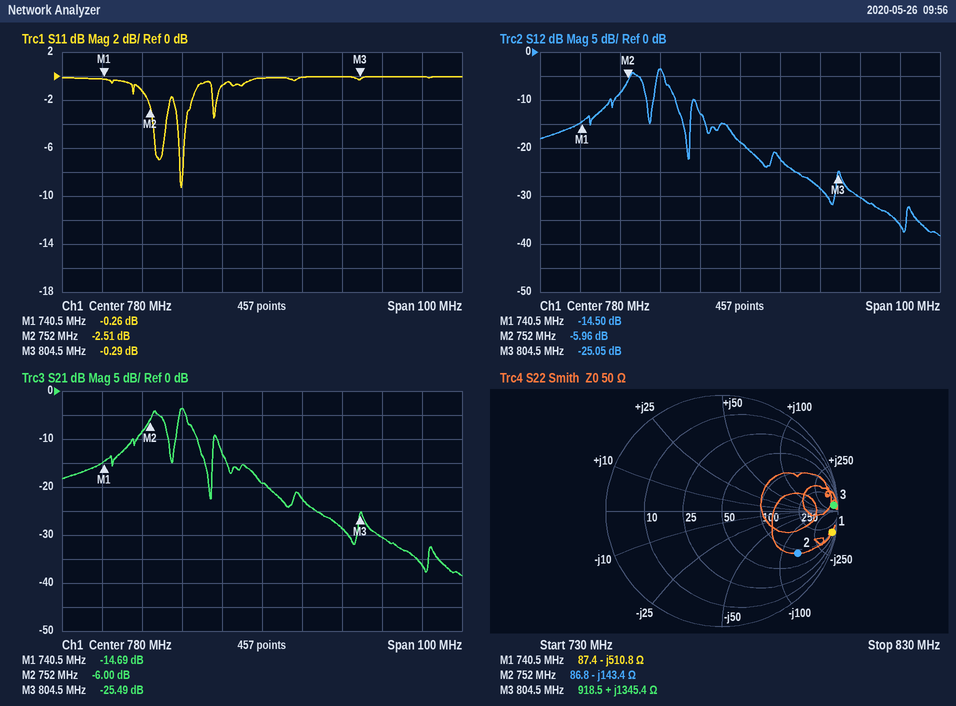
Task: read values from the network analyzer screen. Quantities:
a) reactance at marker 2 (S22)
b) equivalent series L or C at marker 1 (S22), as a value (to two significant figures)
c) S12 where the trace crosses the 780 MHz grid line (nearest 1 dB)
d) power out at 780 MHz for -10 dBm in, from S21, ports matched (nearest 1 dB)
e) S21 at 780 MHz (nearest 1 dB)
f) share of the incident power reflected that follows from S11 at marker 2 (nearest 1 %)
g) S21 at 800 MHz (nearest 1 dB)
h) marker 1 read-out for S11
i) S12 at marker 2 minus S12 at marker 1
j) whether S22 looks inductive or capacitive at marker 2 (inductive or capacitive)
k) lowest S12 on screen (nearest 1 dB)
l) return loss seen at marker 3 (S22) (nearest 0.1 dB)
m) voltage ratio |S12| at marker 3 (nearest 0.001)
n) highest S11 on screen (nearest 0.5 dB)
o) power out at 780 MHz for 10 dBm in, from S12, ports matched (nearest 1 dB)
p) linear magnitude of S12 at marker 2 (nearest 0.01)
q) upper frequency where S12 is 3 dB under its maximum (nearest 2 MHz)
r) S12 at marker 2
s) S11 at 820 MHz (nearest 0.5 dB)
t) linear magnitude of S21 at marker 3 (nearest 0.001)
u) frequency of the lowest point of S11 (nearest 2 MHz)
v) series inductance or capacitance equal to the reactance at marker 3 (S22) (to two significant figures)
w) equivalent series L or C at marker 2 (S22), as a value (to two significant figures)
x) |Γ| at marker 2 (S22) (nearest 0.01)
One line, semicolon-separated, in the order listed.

-143.4 Ω; 420 fF; -19 dB; -29 dBm; -19 dB; 56 %; -29 dB; -0.26 dB; 8.54 dB; capacitive; -38 dB; 0.3 dB; 0.056; 0.0 dB; -9 dBm; 0.50; 762 MHz; -5.96 dB; 0.0 dB; 0.053; 760 MHz; 270 nH; 1.5 pF; 0.75
